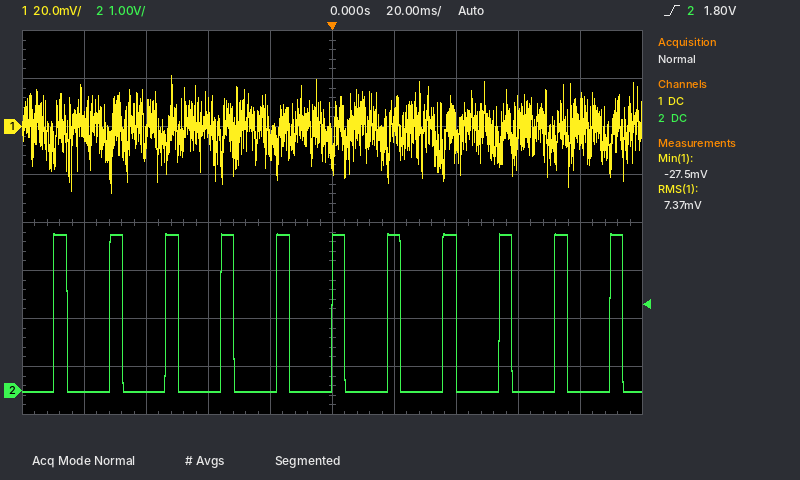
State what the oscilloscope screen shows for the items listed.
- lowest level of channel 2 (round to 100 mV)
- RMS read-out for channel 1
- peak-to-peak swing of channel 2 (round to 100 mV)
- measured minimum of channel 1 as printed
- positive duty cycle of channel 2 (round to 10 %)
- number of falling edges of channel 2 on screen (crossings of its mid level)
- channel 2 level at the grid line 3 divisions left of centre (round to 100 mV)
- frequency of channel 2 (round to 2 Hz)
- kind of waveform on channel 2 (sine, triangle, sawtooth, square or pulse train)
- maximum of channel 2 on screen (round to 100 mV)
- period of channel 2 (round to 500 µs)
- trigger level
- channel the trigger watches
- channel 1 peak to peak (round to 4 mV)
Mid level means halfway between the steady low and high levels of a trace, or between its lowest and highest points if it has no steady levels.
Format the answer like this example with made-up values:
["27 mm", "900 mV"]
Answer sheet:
["0.0 V", "7.37 mV", "3.3 V", "-27.5 mV", "20 %", "11", "0.0 V", "56 Hz", "pulse train", "3.3 V", "18.0 ms", "1.80 V", "channel 2", "48 mV"]
